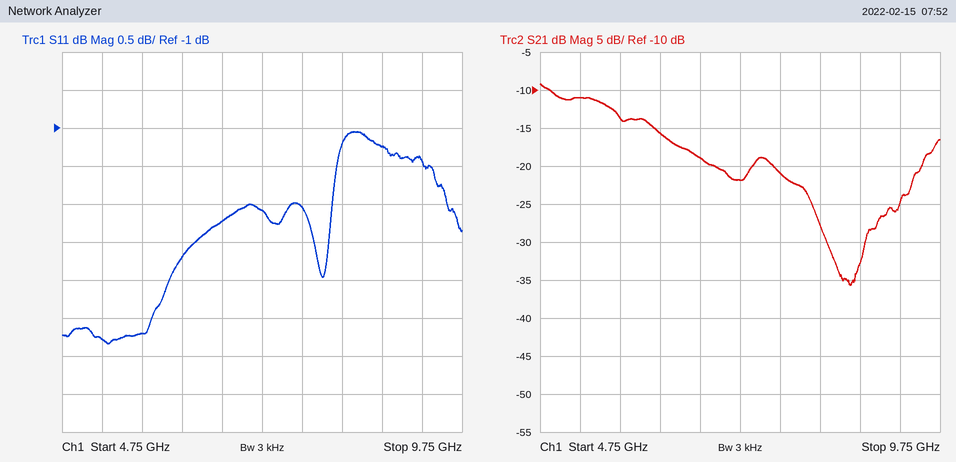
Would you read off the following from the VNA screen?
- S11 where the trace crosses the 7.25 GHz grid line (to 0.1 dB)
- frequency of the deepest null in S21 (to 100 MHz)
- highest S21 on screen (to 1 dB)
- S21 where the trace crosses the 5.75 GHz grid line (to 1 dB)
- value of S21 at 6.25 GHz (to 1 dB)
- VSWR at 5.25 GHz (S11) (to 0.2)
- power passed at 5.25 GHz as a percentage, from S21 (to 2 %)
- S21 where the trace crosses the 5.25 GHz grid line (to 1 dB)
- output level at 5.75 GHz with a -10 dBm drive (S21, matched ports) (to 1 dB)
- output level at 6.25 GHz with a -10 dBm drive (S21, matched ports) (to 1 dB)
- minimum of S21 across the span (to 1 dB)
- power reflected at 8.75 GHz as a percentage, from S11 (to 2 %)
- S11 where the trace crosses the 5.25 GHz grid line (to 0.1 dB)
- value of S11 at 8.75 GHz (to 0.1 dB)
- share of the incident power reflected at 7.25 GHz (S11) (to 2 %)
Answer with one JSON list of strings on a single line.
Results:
["-2.1 dB", "8.6 GHz", "-9 dB", "-14 dB", "-16 dB", "4.6", "8 %", "-11 dB", "-24 dBm", "-26 dBm", "-36 dB", "76 %", "-3.8 dB", "-1.2 dB", "62 %"]
